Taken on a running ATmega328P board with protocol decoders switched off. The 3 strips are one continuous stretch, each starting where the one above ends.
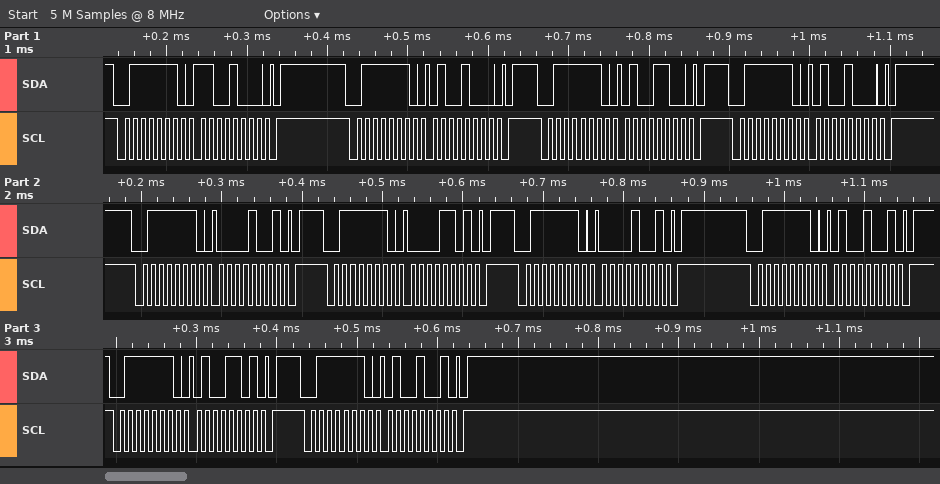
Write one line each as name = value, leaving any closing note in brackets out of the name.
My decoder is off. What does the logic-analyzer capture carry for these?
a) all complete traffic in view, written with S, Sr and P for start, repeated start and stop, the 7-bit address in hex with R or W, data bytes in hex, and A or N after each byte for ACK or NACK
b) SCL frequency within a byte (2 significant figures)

all complete traffic in view, written with S, Sr and P for start, repeated start and stop, the 7-bit address in hex with R or W, data bytes in hex, and A or N after each byte for ACK or NACK = S 3FW A C8 A P S 3FW A 48 A P S 3FW A 4C A P S 3FW A 48 A P S 3FW A 09 A P S 3FW A 0D A P S 3FW A 09 A P S 3FW A 49 A P S 3FW A 4D A P S 3FW A 49 A P
SCL frequency within a byte = 100 kHz
